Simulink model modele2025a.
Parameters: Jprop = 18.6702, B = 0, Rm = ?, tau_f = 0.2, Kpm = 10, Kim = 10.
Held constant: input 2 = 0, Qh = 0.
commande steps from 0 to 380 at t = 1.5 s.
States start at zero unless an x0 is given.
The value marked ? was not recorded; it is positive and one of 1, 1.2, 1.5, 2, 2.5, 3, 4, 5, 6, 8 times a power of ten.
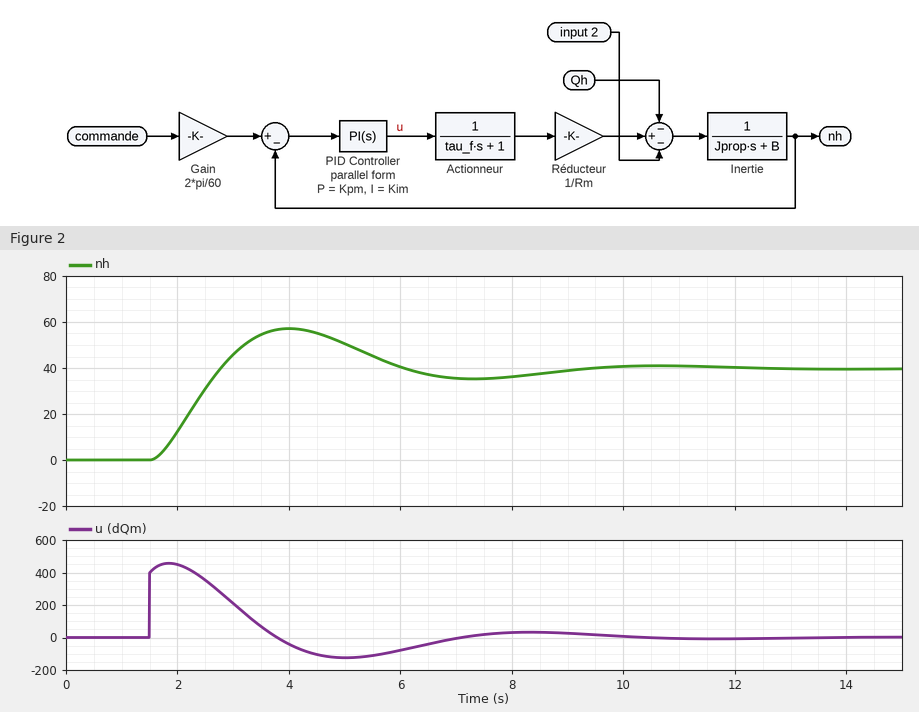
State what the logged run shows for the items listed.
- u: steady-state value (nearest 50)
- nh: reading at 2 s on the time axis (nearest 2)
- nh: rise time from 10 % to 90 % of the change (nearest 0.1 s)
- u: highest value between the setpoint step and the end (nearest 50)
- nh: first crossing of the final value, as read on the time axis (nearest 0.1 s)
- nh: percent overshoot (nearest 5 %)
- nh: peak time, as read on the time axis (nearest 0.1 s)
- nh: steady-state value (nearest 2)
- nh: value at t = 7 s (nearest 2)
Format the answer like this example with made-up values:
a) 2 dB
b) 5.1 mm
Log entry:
a) 0
b) 12
c) 0.9 s
d) 450
e) 2.8 s
f) 45 %
g) 4.0 s
h) 40
i) 36
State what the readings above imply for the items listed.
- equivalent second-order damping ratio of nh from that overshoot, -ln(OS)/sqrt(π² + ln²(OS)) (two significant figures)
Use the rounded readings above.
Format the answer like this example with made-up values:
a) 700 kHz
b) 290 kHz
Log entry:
a) 0.25
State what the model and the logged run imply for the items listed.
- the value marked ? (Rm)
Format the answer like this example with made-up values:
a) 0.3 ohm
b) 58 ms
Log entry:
a) 0.6
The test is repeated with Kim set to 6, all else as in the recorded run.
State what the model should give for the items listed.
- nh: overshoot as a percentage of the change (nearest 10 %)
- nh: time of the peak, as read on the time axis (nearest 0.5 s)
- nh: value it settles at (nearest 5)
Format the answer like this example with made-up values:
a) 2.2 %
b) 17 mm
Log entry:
a) 30 %
b) 4.5 s
c) 40
